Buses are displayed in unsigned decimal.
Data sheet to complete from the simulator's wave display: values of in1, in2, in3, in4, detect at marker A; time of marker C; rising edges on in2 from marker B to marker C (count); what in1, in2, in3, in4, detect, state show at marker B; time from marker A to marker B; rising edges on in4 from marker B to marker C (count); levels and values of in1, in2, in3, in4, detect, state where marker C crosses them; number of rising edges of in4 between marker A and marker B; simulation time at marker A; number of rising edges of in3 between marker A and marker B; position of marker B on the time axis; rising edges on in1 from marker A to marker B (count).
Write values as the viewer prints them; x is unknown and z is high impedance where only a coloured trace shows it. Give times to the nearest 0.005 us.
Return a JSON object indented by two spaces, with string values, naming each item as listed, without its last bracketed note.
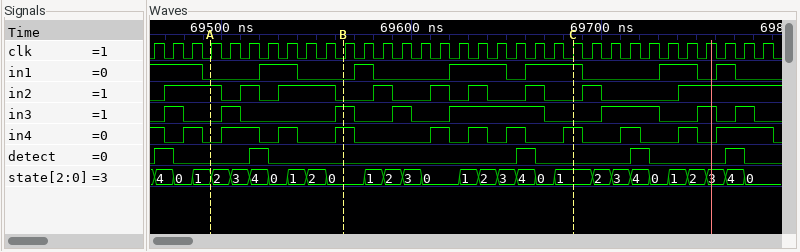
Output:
{
  "values of in1, in2, in3, in4, detect at marker A": "in1=0, in2=1, in3=0, in4=0, detect=0",
  "time of marker C": "69.685 us",
  "rising edges on in2 from marker B to marker C": "4",
  "what in1, in2, in3, in4, detect, state show at marker B": "in1=0, in2=0, in3=1, in4=1, detect=0, state=0",
  "time from marker A to marker B": "0.07 us",
  "rising edges on in4 from marker B to marker C": "4",
  "levels and values of in1, in2, in3, in4, detect, state where marker C crosses them": "in1=1, in2=0, in3=0, in4=1, detect=0, state=1",
  "number of rising edges of in4 between marker A and marker B": "3",
  "simulation time at marker A": "69.495 us",
  "number of rising edges of in3 between marker A and marker B": "2",
  "position of marker B on the time axis": "69.565 us",
  "rising edges on in1 from marker A to marker B": "1"
}
